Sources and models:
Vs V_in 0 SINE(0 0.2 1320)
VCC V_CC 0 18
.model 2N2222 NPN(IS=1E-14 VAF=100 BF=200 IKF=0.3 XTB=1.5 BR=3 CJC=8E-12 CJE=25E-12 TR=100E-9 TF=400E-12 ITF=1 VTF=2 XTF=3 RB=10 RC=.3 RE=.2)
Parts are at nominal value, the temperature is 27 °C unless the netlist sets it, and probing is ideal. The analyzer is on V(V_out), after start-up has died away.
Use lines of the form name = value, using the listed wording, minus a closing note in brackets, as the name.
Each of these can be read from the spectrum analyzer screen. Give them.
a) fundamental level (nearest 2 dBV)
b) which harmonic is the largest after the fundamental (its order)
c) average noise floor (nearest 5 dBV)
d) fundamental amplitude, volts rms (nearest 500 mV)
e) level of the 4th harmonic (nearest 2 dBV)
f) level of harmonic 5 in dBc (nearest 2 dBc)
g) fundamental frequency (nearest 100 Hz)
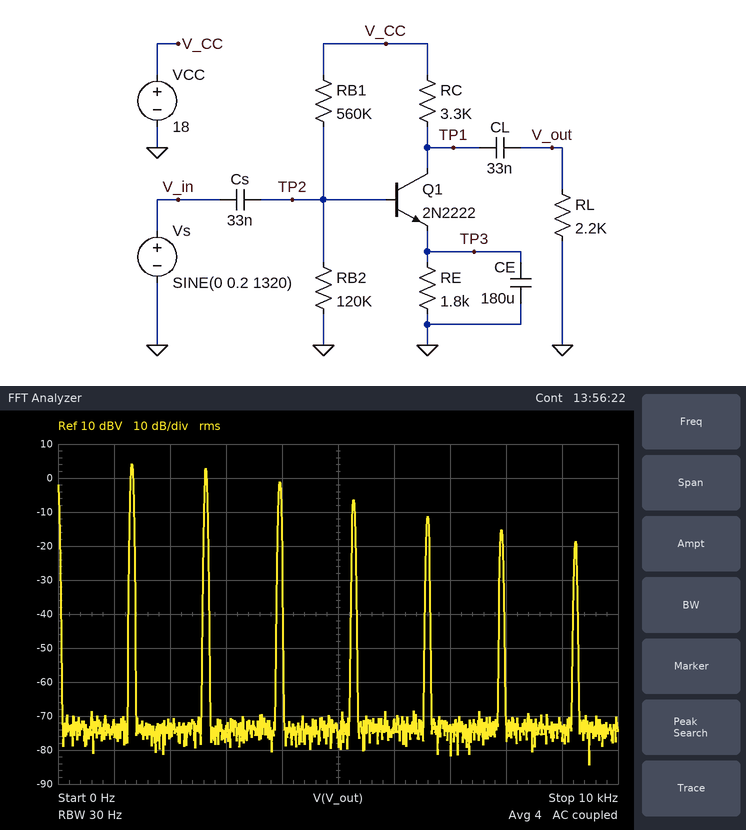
fundamental level = 4 dBV
which harmonic is the largest after the fundamental = 2
average noise floor = -75 dBV
fundamental amplitude, volts rms = 1.5 V
level of the 4th harmonic = -6 dBV
level of harmonic 5 in dBc = -16 dBc
fundamental frequency = 1.3 kHz
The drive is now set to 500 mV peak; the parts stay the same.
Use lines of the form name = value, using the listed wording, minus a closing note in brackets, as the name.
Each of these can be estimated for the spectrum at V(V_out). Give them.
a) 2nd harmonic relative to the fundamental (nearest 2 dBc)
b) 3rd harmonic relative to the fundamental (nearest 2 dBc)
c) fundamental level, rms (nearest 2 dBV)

2nd harmonic relative to the fundamental = 0 dBc
3rd harmonic relative to the fundamental = -2 dBc
fundamental level, rms = 6 dBV
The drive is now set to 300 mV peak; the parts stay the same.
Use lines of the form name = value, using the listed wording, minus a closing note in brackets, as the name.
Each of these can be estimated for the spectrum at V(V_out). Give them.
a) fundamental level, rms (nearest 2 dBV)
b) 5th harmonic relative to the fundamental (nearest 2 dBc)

fundamental level, rms = 4 dBV
5th harmonic relative to the fundamental = -12 dBc
